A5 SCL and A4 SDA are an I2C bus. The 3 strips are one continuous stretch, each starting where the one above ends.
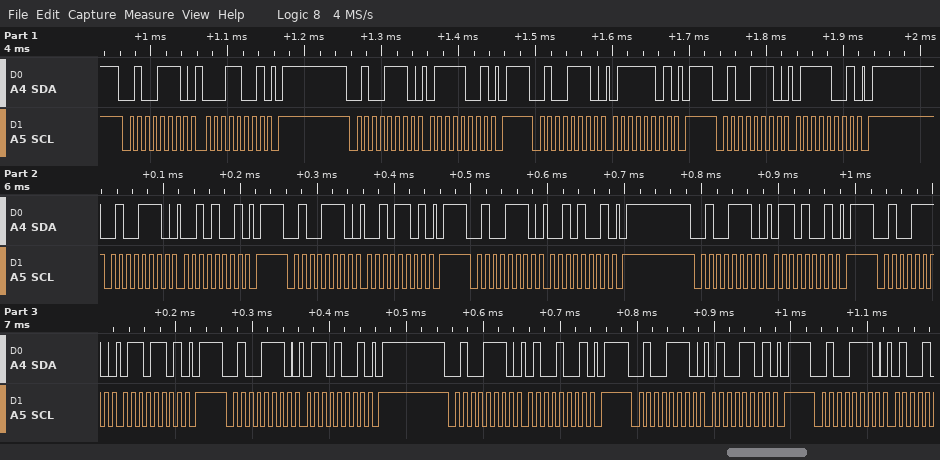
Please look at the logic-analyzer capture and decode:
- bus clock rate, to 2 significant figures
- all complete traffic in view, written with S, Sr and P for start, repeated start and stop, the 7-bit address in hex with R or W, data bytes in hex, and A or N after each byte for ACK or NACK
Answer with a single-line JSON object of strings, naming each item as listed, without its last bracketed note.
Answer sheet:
{"bus clock rate, to 2 significant figures": "100 kHz", "all complete traffic in view, written with S, Sr and P for start, repeated start and stop, the 7-bit address in hex with R or W, data bytes in hex, and A or N after each byte for ACK or NACK": "S 27W A 19 A P S 27W A 79 A P S 27W A 7D A P S 27W A 79 A P S 27W A 29 A P S 27W A 2D A P S 27W A 29 A P S 27W A 69 A P S 27W A 6D A P S 27W A 69 A P S 27W A 49 A P S 27W A 4D A P S 27W A"}
